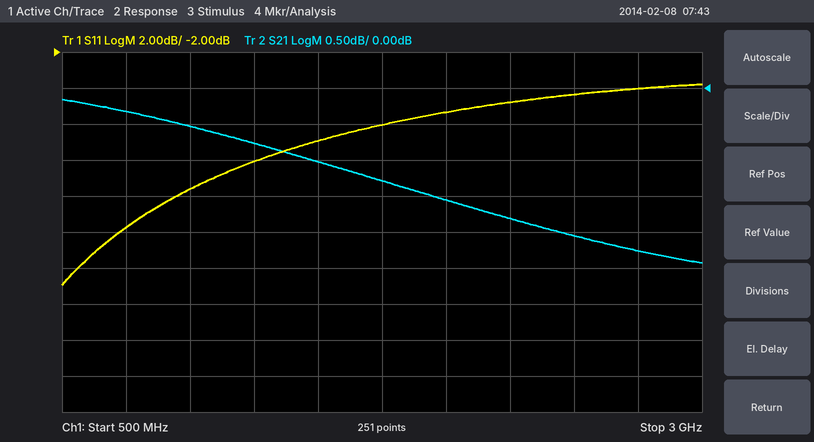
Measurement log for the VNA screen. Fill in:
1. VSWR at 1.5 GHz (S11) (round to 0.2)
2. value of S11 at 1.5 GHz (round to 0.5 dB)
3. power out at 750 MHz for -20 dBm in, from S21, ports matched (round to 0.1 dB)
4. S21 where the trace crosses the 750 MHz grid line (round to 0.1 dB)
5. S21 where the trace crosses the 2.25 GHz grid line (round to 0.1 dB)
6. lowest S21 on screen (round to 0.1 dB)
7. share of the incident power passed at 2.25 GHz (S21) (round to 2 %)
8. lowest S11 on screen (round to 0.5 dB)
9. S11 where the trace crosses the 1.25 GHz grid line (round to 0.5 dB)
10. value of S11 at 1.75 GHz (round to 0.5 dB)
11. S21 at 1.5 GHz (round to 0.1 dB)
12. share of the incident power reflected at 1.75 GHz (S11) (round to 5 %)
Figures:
2.6
-7.0 dB
-20.3 dBm
-0.3 dB
-1.8 dB
-2.4 dB
66 %
-15.0 dB
-8.0 dB
-6.0 dB
-1.0 dB
25 %
